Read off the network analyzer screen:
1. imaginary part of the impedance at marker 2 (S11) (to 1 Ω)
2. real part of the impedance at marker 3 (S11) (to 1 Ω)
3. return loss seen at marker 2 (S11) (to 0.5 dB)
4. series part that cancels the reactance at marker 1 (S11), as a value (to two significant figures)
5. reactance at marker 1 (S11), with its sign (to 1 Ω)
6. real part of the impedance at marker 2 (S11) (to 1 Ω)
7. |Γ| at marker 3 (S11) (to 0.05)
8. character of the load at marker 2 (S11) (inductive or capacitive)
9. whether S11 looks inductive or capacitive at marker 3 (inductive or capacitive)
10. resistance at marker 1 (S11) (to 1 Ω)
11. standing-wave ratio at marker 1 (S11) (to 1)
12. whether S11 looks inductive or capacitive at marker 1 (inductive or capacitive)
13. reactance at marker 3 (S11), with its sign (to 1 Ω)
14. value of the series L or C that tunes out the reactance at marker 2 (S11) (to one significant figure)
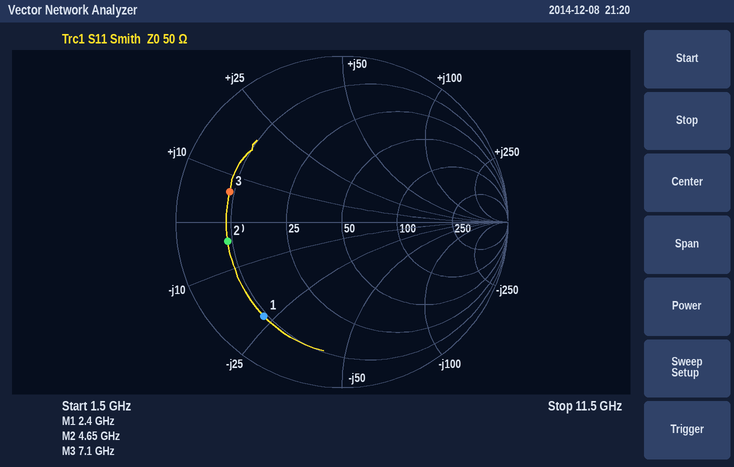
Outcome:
-4 Ω
9 Ω
3.0 dB
1.5 nH
-23 Ω
9 Ω
0.70
capacitive
inductive
9 Ω
7
capacitive
+6 Ω
100 pH
